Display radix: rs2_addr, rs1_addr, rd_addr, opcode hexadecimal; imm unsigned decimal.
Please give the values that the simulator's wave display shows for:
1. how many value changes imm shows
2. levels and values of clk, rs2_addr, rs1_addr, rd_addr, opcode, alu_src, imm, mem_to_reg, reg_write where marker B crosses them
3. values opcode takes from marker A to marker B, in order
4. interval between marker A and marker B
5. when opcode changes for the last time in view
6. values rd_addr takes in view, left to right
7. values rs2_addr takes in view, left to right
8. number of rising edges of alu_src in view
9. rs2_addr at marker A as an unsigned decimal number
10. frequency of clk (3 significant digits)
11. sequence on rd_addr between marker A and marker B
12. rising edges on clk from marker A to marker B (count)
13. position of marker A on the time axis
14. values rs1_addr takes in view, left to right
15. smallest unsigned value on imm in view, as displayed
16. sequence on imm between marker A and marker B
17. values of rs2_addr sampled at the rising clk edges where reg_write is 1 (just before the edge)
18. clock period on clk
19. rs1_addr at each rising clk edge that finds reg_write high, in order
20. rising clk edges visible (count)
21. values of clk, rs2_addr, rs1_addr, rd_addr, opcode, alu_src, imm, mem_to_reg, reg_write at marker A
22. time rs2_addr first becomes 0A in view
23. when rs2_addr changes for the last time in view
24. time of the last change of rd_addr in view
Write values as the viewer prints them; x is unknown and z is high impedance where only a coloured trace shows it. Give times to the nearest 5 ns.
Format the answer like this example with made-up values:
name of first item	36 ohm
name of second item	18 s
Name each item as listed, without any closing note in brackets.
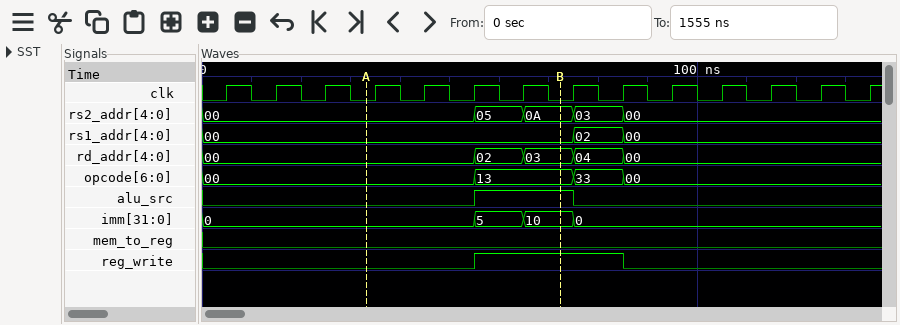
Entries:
how many value changes imm shows	3
levels and values of clk, rs2_addr, rs1_addr, rd_addr, opcode, alu_src, imm, mem_to_reg, reg_write where marker B crosses them	clk=0, rs2_addr=0A, rs1_addr=00, rd_addr=03, opcode=13, alu_src=1, imm=10, mem_to_reg=0, reg_write=1
values opcode takes from marker A to marker B, in order	00, 13
interval between marker A and marker B	40 ns
when opcode changes for the last time in view	85 ns
values rd_addr takes in view, left to right	00, 02, 03, 04, 00
values rs2_addr takes in view, left to right	00, 05, 0A, 03, 00
number of rising edges of alu_src in view	1
rs2_addr at marker A as an unsigned decimal number	0
frequency of clk	100 MHz
sequence on rd_addr between marker A and marker B	00, 02, 03
rising edges on clk from marker A to marker B	4
position of marker A on the time axis	35 ns
values rs1_addr takes in view, left to right	00, 02, 00
smallest unsigned value on imm in view, as displayed	0
sequence on imm between marker A and marker B	0, 5, 10
values of rs2_addr sampled at the rising clk edges where reg_write is 1	05, 0A, 03
clock period on clk	10 ns
rs1_addr at each rising clk edge that finds reg_write high, in order	00, 00, 02
rising clk edges visible	14
values of clk, rs2_addr, rs1_addr, rd_addr, opcode, alu_src, imm, mem_to_reg, reg_write at marker A	clk=0, rs2_addr=00, rs1_addr=00, rd_addr=00, opcode=00, alu_src=0, imm=0, mem_to_reg=0, reg_write=0
time rs2_addr first becomes 0A in view	65 ns
when rs2_addr changes for the last time in view	85 ns
time of the last change of rd_addr in view	85 ns
